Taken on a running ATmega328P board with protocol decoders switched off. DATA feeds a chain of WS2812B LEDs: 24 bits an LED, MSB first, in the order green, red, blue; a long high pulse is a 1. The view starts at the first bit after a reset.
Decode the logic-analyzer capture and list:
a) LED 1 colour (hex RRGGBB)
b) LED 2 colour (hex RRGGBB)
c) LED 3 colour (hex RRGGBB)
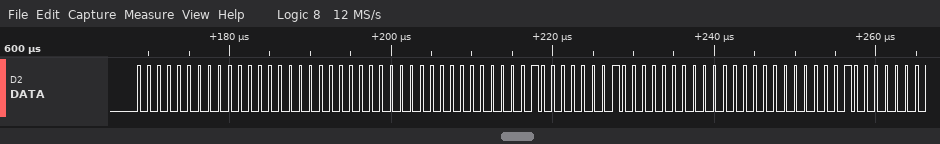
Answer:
#000000
#010001
#000002
